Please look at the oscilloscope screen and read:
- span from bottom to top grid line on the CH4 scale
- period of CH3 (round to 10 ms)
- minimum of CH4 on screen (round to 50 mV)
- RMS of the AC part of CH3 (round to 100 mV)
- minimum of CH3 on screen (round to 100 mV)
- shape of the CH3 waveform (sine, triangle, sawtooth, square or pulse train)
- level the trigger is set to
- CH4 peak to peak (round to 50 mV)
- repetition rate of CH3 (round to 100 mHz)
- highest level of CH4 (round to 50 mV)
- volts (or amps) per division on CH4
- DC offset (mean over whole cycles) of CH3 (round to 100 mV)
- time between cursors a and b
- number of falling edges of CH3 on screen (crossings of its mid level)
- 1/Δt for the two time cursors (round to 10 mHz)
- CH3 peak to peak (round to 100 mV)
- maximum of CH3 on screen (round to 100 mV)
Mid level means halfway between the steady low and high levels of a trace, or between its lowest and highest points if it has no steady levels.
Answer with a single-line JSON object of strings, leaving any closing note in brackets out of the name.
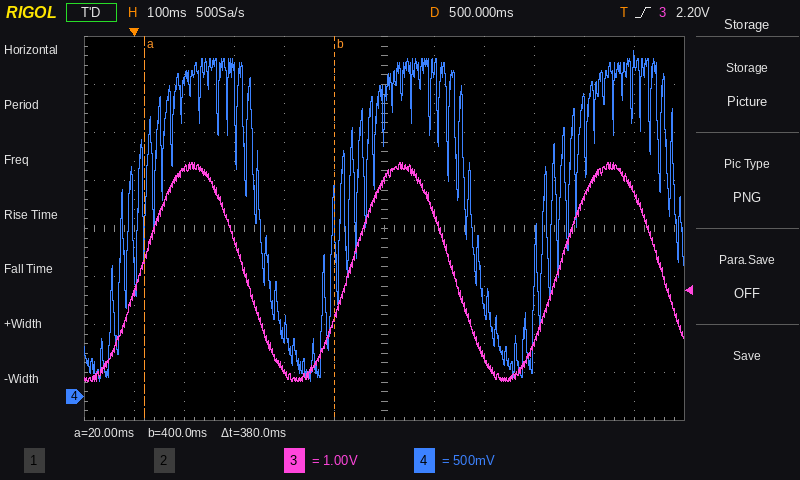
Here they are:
{"span from bottom to top grid line on the CH4 scale": "4 V", "period of CH3": "420 ms", "minimum of CH4 on screen": "150 mV", "RMS of the AC part of CH3": "1.6 V", "minimum of CH3 on screen": "300 mV", "shape of the CH3 waveform": "sine", "level the trigger is set to": "2.20 V", "CH4 peak to peak": "3.45 V", "repetition rate of CH3": "2.4 Hz", "highest level of CH4": "3.60 V", "volts (or amps) per division on CH4": "500 mV", "DC offset (mean over whole cycles) of CH3": "2.6 V", "time between cursors a and b": "380 ms", "number of falling edges of CH3 on screen": "3", "1/Δt for the two time cursors": "2.63 Hz", "CH3 peak to peak": "4.6 V", "maximum of CH3 on screen": "4.9 V"}
